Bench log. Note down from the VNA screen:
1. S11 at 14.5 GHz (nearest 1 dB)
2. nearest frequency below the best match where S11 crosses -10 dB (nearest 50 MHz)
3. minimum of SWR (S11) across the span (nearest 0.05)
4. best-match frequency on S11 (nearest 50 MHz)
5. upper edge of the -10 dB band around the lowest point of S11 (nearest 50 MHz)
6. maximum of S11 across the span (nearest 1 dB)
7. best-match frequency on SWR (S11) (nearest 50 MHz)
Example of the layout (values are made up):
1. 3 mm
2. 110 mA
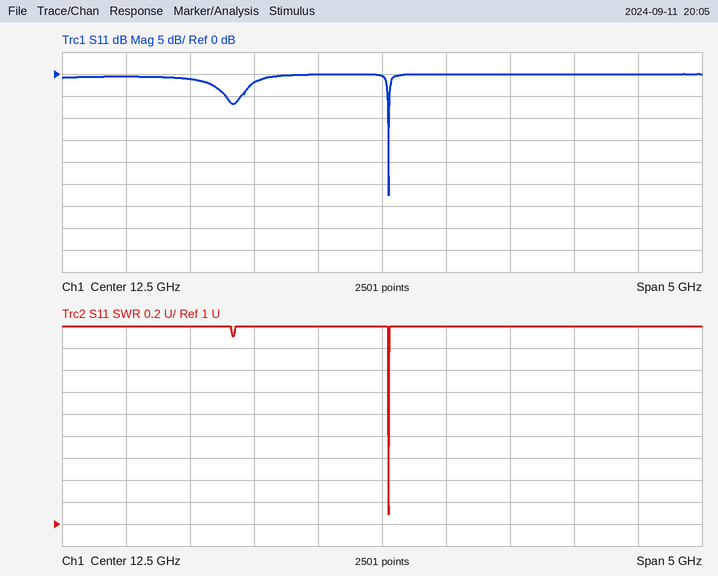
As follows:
1. 0 dB
2. 12.55 GHz
3. 1.10
4. 12.55 GHz
5. 12.55 GHz
6. 0 dB
7. 12.55 GHz
